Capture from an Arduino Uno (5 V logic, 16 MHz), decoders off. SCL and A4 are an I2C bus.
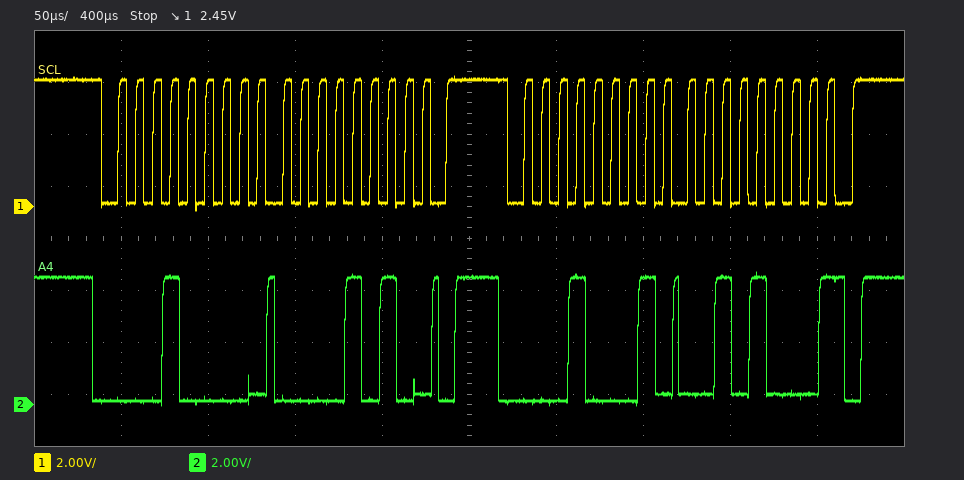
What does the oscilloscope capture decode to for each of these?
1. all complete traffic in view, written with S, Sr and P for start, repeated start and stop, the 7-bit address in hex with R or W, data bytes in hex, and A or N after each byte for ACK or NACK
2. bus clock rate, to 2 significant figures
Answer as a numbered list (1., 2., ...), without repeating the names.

1. S 08W A 0A A P S 08R A 28 N P
2. 100 kHz
